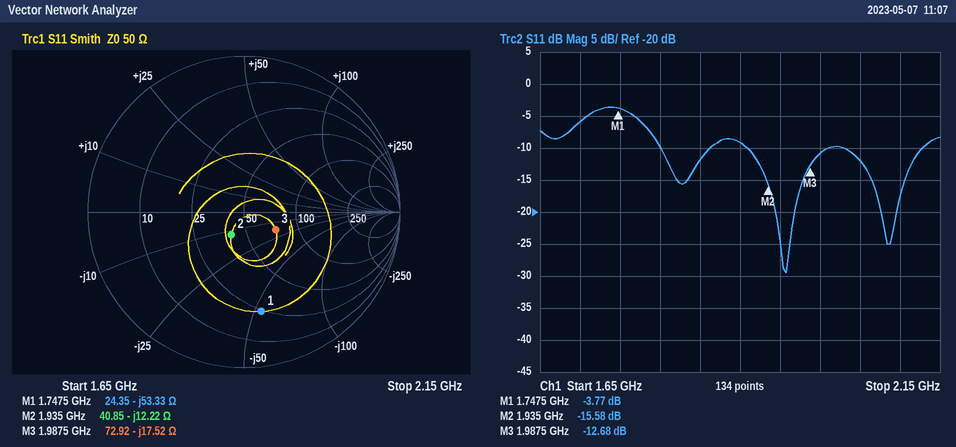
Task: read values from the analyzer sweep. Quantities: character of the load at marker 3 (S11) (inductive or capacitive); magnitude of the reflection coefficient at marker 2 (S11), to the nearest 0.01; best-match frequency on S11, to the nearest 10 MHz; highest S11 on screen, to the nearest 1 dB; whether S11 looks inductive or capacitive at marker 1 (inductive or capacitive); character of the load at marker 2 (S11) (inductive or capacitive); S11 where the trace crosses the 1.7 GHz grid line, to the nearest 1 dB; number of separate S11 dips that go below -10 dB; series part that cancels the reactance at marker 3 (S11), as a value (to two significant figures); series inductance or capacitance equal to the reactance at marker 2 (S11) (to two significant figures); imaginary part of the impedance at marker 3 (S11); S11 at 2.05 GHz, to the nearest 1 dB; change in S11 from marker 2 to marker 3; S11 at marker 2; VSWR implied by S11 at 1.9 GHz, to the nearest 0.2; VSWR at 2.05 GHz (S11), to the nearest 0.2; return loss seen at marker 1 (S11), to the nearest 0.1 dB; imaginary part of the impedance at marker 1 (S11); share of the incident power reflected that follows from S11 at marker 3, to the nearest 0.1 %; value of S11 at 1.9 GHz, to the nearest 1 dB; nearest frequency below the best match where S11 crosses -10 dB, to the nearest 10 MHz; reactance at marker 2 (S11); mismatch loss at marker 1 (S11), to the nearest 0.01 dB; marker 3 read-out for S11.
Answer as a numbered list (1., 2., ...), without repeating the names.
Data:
1. capacitive
2. 0.17
3. 1.96 GHz
4. -4 dB
5. capacitive
6. capacitive
7. -6 dB
8. 3
9. 1.4 nH
10. 6.7 pF
11. -17.52 Ω
12. -12 dB
13. 2.90 dB
14. -15.58 dB
15. 2.0
16. 1.6
17. 3.8 dB
18. -53.33 Ω
19. 5.4 %
20. -9 dB
21. 1.91 GHz
22. -12.22 Ω
23. 2.36 dB
24. -12.68 dB
